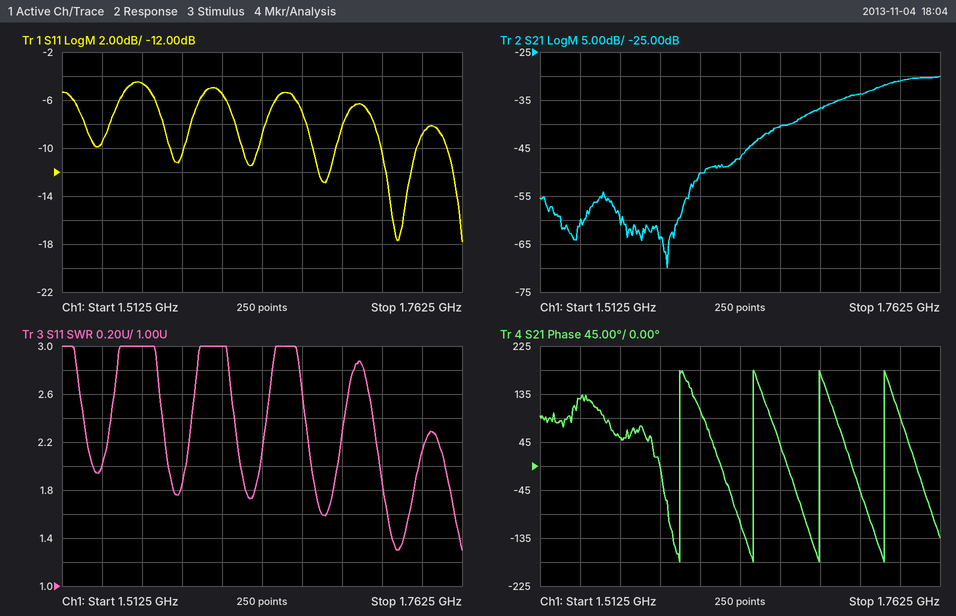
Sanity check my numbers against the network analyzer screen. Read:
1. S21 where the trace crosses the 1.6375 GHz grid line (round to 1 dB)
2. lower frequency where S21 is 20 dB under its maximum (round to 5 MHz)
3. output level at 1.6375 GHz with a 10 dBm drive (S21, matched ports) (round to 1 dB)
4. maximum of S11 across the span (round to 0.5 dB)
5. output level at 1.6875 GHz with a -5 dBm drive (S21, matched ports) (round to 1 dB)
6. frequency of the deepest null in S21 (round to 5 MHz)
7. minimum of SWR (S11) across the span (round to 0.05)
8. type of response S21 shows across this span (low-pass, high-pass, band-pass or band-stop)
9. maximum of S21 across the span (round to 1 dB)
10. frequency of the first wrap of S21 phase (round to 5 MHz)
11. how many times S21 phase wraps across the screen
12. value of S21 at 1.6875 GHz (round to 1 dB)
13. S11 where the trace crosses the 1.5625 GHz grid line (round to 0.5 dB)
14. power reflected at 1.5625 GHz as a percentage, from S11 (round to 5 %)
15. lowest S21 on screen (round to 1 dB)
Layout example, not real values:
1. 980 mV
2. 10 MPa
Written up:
1. -47 dB
2. 1.615 GHz
3. -37 dBm
4. -4.5 dB
5. -42 dBm
6. 1.590 GHz
7. 1.30
8. high-pass
9. -30 dB
10. 1.600 GHz
11. 4
12. -37 dB
13. -4.5 dB
14. 35 %
15. -70 dB
